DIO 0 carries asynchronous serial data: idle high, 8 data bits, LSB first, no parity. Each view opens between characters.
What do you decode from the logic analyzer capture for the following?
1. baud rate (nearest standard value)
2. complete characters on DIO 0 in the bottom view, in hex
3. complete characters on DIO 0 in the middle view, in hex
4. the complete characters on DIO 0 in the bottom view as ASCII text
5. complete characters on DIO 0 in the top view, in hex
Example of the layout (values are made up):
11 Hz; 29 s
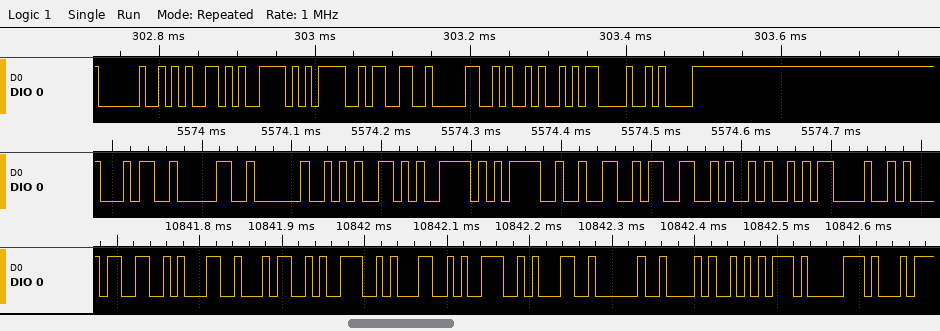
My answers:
115200 baud; 33, 31, 34, 39, 31, 39, 31, 20, 28, 75, 70; 34, 30, 20, 65, 79, 3D, 32, 33, 29, 0D; "3149191 (up"; 20, 65, 79, 3D, 33, 30, 29, 0D, 0A
